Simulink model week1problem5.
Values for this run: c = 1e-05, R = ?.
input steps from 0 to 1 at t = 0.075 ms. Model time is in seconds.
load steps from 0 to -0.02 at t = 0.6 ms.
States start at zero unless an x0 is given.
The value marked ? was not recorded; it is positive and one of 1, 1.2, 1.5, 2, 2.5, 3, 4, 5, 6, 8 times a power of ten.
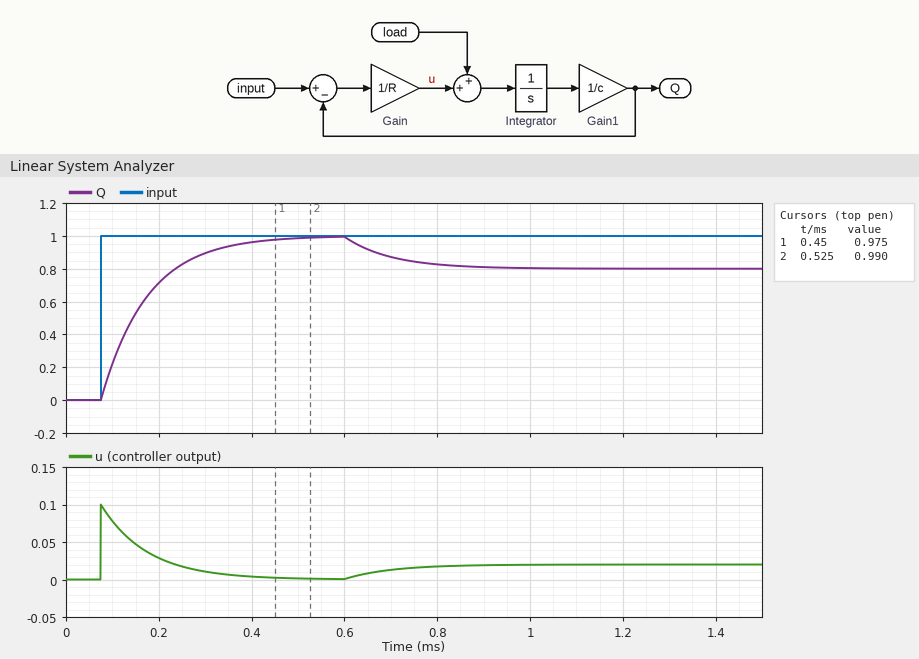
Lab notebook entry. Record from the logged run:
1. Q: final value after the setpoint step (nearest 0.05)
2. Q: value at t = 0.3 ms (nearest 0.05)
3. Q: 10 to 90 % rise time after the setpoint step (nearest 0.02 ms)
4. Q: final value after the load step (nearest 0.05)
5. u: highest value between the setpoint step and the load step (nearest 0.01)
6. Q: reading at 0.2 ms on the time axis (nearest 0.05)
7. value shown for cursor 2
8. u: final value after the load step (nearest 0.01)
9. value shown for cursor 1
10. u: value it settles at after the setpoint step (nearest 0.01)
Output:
1.00
0.90
0.22 ms
0.80
0.10
0.70
0.990
0.02
0.975
0.00
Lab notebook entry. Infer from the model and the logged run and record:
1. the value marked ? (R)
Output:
10
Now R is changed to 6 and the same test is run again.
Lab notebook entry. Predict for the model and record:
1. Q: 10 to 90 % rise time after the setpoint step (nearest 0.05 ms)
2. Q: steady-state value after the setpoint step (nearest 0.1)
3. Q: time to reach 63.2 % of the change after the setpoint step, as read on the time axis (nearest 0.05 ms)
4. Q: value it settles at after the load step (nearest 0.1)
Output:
0.15 ms
1.0
0.15 ms
0.9
